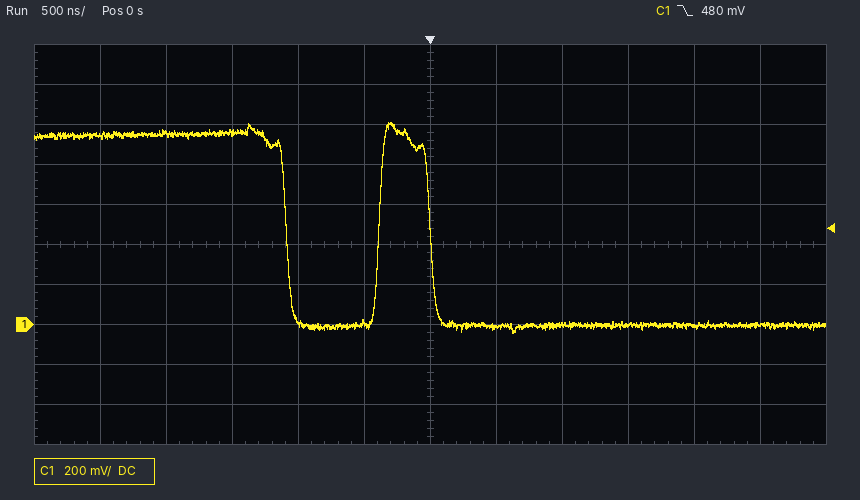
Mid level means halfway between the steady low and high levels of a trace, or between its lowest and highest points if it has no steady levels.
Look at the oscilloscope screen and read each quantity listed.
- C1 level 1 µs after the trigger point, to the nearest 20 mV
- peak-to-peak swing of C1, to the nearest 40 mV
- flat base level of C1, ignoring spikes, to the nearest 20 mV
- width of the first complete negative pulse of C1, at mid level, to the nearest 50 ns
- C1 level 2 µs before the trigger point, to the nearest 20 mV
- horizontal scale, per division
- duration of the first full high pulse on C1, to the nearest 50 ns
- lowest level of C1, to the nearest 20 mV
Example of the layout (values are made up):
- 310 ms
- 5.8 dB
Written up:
- 0 mV
- 1.04 V
- 0 mV
- 700 ns
- 960 mV
- 500 ns
- 400 ns
- -40 mV
